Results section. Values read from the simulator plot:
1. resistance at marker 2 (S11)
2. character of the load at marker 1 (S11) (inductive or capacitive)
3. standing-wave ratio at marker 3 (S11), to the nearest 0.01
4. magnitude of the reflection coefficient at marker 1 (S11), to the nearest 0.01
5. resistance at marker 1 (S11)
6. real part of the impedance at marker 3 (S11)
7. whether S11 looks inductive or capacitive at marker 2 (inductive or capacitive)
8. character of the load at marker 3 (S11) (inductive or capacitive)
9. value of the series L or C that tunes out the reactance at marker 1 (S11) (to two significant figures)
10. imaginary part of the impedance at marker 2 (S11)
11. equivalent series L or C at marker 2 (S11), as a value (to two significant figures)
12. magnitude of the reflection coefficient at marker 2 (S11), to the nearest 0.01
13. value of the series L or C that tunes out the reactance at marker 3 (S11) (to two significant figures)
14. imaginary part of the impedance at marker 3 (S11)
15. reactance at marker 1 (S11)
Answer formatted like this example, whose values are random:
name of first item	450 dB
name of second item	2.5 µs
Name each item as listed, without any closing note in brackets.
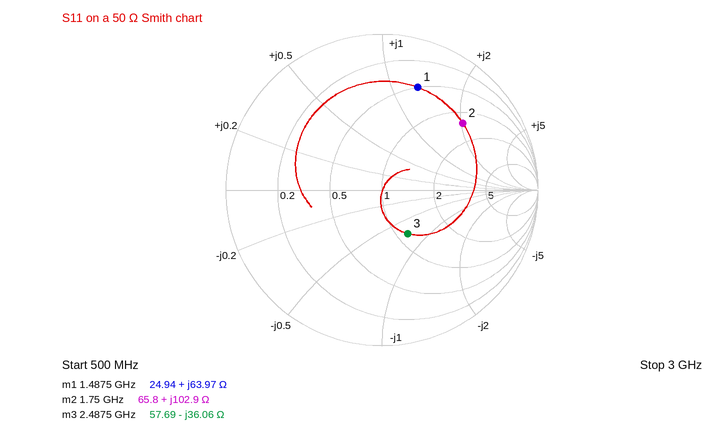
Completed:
resistance at marker 2	65.8 Ω
character of the load at marker 1 (S11)	inductive
standing-wave ratio at marker 3 (S11), to the nearest 0.01	1.96
magnitude of the reflection coefficient at marker 1 (S11), to the nearest 0.01	0.70
resistance at marker 1	24.94 Ω
real part of the impedance at marker 3	57.69 Ω
whether S11 looks inductive or capacitive at marker 2	inductive
character of the load at marker 3 (S11)	capacitive
value of the series L or C that tunes out the reactance at marker 1 (S11)	1.7 pF
imaginary part of the impedance at marker 2	+102.9 Ω
equivalent series L or C at marker 2 (S11), as a value	9.4 nH
magnitude of the reflection coefficient at marker 2 (S11), to the nearest 0.01	0.67
value of the series L or C that tunes out the reactance at marker 3 (S11)	2.3 nH
imaginary part of the impedance at marker 3	-36.06 Ω
reactance at marker 1	+63.97 Ω
